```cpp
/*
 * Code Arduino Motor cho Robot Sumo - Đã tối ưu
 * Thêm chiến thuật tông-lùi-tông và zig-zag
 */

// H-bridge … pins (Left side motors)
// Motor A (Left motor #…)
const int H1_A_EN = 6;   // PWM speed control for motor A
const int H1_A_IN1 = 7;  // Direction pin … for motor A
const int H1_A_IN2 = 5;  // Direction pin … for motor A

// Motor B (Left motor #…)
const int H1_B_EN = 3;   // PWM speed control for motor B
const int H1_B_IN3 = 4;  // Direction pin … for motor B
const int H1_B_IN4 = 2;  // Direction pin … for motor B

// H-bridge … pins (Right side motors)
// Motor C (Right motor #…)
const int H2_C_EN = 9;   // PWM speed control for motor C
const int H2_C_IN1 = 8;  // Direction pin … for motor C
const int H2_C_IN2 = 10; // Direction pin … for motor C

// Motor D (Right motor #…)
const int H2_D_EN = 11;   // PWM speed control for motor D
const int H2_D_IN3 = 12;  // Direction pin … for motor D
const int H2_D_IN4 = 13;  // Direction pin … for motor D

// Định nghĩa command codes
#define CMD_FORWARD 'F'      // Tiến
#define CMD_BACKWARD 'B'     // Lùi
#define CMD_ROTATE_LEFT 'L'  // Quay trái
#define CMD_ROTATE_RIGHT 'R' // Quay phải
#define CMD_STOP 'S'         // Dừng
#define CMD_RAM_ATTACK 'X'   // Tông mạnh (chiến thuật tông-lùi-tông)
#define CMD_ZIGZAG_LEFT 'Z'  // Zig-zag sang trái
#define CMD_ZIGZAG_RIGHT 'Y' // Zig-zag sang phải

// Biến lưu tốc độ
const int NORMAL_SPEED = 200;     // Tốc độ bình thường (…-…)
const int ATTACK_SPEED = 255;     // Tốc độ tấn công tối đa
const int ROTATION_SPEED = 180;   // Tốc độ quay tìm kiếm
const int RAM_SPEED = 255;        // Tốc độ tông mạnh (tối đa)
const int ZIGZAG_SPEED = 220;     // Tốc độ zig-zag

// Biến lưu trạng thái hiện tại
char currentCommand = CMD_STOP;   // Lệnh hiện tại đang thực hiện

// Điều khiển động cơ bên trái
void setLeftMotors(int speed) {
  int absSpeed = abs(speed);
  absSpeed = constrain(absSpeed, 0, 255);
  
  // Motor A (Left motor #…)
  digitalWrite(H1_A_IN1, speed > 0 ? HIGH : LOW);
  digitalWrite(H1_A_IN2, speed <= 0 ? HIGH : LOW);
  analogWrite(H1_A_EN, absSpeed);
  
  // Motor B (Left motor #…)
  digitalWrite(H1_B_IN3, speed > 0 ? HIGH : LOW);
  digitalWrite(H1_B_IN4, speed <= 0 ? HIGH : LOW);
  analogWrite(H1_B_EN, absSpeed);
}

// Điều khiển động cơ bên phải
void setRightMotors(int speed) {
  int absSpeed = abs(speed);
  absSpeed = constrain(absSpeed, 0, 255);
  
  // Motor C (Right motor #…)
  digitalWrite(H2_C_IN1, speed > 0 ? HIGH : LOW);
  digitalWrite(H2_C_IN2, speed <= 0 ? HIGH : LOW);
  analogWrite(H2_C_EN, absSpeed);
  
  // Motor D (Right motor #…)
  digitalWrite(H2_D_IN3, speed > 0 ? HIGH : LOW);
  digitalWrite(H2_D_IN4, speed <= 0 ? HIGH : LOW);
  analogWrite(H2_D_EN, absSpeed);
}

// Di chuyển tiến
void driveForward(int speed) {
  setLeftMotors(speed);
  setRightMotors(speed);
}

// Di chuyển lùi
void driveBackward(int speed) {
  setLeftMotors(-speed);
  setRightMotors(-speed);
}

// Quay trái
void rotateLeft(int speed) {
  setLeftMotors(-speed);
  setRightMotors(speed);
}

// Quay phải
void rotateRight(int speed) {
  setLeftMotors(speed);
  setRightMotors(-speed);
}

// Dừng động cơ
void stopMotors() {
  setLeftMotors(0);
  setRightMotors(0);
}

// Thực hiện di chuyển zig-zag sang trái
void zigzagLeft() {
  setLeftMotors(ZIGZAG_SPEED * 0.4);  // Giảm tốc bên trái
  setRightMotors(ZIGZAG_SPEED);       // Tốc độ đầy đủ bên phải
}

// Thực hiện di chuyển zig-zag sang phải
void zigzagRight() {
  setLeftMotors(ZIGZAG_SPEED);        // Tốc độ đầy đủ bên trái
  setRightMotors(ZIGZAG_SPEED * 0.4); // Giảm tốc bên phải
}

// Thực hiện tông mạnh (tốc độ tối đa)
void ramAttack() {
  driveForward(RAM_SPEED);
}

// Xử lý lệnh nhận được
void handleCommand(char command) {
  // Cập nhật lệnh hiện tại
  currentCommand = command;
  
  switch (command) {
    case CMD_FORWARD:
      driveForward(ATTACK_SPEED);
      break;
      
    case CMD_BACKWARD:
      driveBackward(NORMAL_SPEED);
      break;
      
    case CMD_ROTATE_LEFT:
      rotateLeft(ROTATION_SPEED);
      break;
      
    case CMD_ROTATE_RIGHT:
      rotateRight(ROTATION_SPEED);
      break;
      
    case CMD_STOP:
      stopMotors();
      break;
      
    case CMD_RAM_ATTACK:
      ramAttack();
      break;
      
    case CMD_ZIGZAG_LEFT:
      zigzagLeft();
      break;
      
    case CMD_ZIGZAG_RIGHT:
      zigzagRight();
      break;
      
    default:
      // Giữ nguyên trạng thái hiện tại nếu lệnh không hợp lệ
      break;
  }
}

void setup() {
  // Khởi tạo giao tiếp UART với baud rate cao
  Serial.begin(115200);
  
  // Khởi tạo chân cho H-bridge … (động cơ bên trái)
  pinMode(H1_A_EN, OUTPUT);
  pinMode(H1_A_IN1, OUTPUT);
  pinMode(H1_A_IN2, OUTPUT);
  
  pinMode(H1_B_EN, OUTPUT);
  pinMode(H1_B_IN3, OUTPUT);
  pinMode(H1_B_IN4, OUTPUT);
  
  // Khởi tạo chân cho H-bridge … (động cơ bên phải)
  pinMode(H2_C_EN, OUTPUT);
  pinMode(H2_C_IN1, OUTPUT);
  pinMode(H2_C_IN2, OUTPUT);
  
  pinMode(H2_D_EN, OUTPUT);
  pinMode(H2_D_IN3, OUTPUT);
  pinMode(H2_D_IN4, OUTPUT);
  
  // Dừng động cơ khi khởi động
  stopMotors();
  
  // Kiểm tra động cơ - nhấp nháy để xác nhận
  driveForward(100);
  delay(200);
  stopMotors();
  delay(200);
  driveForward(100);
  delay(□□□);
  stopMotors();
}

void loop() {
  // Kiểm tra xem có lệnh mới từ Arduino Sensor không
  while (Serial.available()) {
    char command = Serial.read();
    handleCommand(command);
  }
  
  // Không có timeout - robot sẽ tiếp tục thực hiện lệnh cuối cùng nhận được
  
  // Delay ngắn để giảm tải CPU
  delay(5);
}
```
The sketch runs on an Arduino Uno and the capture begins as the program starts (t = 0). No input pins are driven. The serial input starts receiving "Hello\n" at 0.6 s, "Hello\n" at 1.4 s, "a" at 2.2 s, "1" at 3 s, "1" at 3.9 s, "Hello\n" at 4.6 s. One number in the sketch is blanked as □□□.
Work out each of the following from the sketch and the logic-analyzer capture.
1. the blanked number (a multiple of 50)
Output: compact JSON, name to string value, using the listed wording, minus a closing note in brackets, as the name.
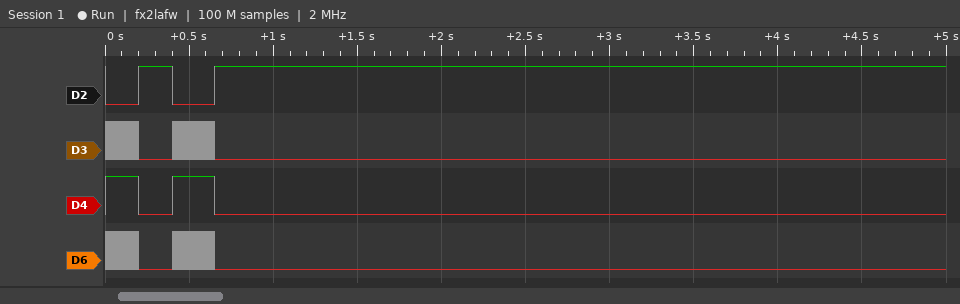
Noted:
{"the blanked number": "250"}
